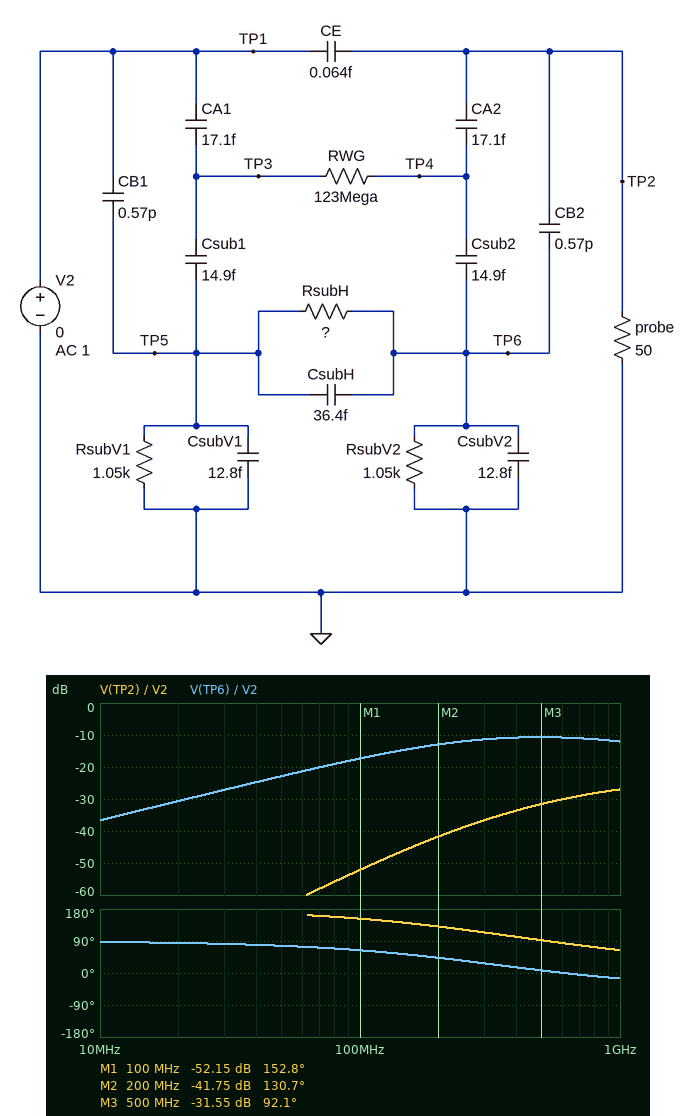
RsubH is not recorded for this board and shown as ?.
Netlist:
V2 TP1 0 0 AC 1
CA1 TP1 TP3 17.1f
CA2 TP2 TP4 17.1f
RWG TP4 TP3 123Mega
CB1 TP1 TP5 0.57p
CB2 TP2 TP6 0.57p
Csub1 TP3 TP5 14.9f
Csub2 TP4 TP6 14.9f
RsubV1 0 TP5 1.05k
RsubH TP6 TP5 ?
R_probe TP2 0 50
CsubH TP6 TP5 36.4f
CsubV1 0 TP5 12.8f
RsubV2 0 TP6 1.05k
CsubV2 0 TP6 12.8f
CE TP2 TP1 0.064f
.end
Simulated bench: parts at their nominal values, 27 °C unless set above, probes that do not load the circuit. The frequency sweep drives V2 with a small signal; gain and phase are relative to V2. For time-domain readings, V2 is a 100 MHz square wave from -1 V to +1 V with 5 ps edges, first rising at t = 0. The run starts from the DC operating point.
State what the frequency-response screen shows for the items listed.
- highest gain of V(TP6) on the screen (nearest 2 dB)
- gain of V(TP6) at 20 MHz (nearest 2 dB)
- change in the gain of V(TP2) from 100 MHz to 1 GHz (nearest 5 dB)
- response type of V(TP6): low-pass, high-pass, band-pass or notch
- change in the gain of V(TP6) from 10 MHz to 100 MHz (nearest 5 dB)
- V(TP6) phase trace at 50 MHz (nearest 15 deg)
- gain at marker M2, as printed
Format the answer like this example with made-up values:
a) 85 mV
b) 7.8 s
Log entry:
a) -10 dB
b) -30 dB
c) 25 dB
d) high-pass
e) 20 dB
f) 75 deg
g) -41.75 dB
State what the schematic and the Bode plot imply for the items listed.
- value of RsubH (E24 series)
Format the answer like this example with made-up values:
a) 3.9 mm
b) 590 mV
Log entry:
a) 620 Ω
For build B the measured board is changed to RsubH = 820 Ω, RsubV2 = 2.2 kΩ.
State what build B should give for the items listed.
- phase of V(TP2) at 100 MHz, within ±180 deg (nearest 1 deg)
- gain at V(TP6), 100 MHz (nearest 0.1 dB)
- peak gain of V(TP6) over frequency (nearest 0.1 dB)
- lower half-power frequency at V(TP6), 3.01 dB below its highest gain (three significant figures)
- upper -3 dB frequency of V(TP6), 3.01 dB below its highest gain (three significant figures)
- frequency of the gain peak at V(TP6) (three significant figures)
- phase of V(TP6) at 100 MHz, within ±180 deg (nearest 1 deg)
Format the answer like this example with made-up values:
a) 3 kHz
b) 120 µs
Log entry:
a) 144 deg
b) -15.0 dB
c) -10.5 dB
d) 127 MHz
e) 1.09 GHz
f) 366 MHz
g) 55 deg
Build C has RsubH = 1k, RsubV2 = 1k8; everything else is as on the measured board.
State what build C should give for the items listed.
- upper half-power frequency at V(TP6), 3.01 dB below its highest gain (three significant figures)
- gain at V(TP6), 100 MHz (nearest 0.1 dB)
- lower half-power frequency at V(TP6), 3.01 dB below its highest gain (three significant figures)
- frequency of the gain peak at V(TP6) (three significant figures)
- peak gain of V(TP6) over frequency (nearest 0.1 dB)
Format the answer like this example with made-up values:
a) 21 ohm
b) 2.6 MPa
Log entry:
a) 1.02 GHz
b) -16.1 dB
c) 130 MHz
d) 357 MHz
e) -11.5 dB
